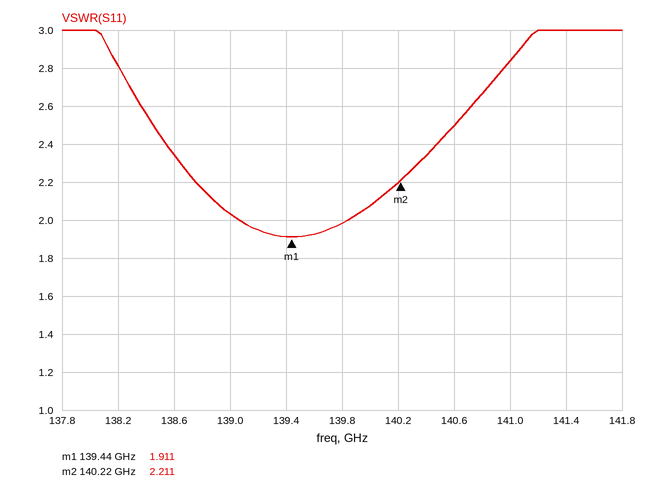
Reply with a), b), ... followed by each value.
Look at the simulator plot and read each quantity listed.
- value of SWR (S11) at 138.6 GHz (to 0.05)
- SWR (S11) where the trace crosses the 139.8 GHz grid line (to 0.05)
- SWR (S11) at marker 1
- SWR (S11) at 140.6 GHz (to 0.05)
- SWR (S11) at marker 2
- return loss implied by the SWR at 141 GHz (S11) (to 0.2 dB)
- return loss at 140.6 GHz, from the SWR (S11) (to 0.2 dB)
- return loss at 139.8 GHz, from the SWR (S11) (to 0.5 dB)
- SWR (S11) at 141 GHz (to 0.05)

a) 2.35
b) 2.00
c) 1.911
d) 2.50
e) 2.211
f) 6.4 dB
g) 7.4 dB
h) 9.5 dB
i) 2.85
